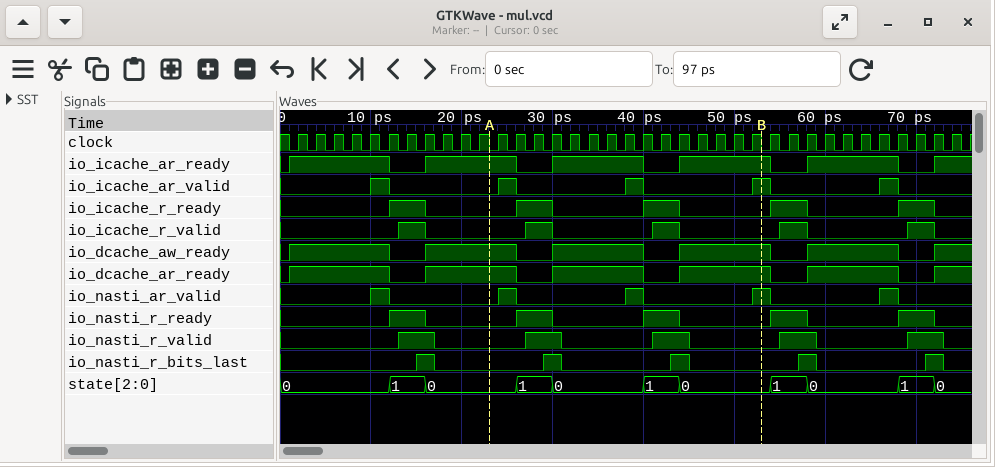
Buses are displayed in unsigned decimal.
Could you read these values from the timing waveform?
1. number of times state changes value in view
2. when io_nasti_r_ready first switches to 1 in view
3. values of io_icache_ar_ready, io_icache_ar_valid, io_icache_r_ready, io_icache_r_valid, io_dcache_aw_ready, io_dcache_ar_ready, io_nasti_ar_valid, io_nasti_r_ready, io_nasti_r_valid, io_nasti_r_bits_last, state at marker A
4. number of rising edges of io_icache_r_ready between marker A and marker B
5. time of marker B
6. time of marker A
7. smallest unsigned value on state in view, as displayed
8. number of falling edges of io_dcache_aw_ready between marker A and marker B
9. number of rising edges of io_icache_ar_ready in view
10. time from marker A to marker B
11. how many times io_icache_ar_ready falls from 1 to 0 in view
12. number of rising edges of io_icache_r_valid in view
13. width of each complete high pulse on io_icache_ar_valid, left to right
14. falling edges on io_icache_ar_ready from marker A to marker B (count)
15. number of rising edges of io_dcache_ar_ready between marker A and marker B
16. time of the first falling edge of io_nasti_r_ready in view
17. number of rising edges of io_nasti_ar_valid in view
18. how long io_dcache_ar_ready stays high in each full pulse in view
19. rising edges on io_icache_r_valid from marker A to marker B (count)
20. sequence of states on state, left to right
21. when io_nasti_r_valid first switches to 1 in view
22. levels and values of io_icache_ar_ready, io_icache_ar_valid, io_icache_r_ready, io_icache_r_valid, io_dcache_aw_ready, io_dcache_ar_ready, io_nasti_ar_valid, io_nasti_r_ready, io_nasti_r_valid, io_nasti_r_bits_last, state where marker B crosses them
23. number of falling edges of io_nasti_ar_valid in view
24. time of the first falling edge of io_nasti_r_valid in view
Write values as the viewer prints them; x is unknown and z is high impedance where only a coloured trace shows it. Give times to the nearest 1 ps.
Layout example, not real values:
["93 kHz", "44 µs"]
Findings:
["10", "12 ps", "io_icache_ar_ready=1, io_icache_ar_valid=0, io_icache_r_ready=0, io_icache_r_valid=0, io_dcache_aw_ready=1, io_dcache_ar_ready=1, io_nasti_ar_valid=0, io_nasti_r_ready=0, io_nasti_r_valid=0, io_nasti_r_bits_last=0, state=0", "2", "53 ps", "23 ps", "0", "2", "6", "30 ps", "5", "5", "2 ps, 2 ps, 2 ps, 2 ps, 2 ps", "2", "2", "16 ps", "5", "11 ps, 10 ps, 10 ps, 10 ps, 10 ps", "2", "0, 1, 0, 1, 0, 1, 0, 1, 0, 1, 0", "13 ps", "io_icache_ar_ready=1, io_icache_ar_valid=1, io_icache_r_ready=0, io_icache_r_valid=0, io_dcache_aw_ready=1, io_dcache_ar_ready=1, io_nasti_ar_valid=1, io_nasti_r_ready=0, io_nasti_r_valid=0, io_nasti_r_bits_last=0, state=0", "5", "17 ps"]
